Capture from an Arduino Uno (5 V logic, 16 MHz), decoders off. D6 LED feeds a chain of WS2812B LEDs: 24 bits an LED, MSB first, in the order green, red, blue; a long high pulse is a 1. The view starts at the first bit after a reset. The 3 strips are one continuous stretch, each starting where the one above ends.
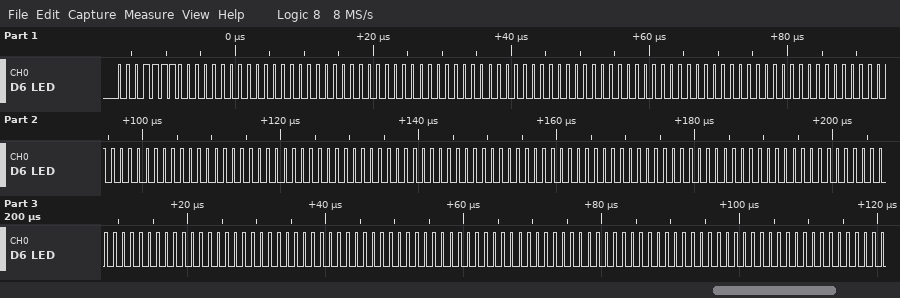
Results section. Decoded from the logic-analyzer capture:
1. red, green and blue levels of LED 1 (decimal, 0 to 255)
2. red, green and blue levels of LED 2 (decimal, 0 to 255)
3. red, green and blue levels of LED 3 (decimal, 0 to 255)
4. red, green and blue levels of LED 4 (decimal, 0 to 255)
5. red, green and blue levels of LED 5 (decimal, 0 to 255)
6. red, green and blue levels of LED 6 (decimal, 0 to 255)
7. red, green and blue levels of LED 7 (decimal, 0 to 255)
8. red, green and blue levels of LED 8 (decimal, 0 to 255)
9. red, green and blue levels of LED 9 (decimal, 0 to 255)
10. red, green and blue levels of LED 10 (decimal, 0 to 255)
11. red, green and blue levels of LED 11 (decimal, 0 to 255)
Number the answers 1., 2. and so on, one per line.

1. 0, 30, 0
2. 0, 0, 0
3. 0, 0, 0
4. 0, 0, 0
5. 0, 0, 0
6. 0, 0, 0
7. 0, 0, 0
8. 0, 0, 0
9. 0, 0, 0
10. 0, 0, 0
11. 0, 0, 0
